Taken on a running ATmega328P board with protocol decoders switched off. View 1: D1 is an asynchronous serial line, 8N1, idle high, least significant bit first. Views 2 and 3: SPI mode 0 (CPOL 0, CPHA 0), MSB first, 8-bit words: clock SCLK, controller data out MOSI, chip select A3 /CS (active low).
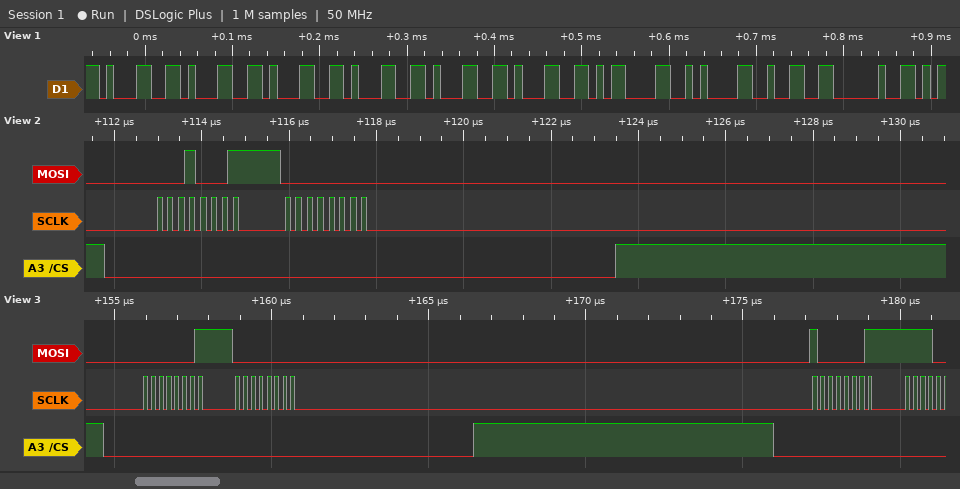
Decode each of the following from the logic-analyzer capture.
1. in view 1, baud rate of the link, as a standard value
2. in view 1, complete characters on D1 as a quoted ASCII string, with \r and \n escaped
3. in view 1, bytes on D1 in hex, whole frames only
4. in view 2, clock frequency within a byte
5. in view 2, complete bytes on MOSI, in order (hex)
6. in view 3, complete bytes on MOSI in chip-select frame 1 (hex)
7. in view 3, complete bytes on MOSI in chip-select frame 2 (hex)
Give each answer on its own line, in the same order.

115200 baud
"111111\r\n2 "
31 31 31 31 31 31 0D 0A 32 20
4 MHz
11 00
01 00
81
